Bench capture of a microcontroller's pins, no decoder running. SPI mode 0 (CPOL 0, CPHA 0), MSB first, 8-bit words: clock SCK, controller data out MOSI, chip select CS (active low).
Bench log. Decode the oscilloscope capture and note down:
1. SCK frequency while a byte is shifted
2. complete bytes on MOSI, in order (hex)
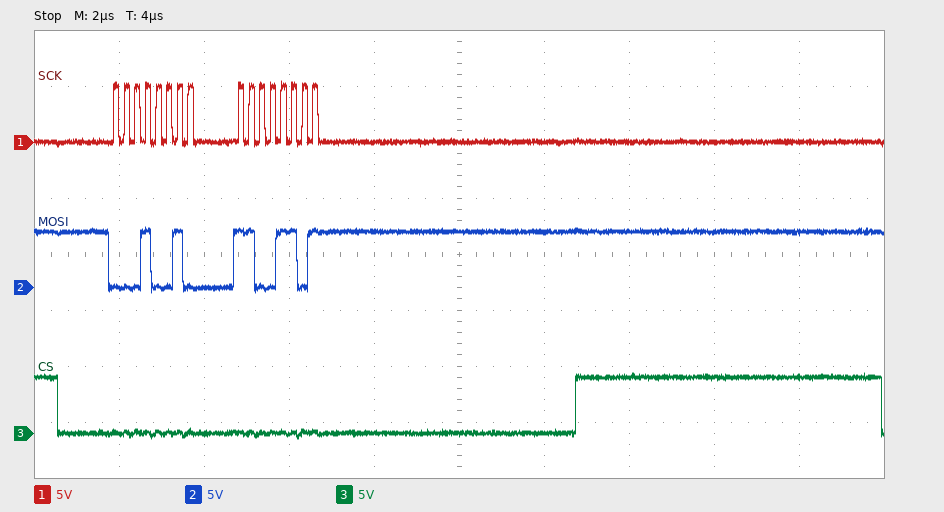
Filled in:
4 MHz
12 CD
